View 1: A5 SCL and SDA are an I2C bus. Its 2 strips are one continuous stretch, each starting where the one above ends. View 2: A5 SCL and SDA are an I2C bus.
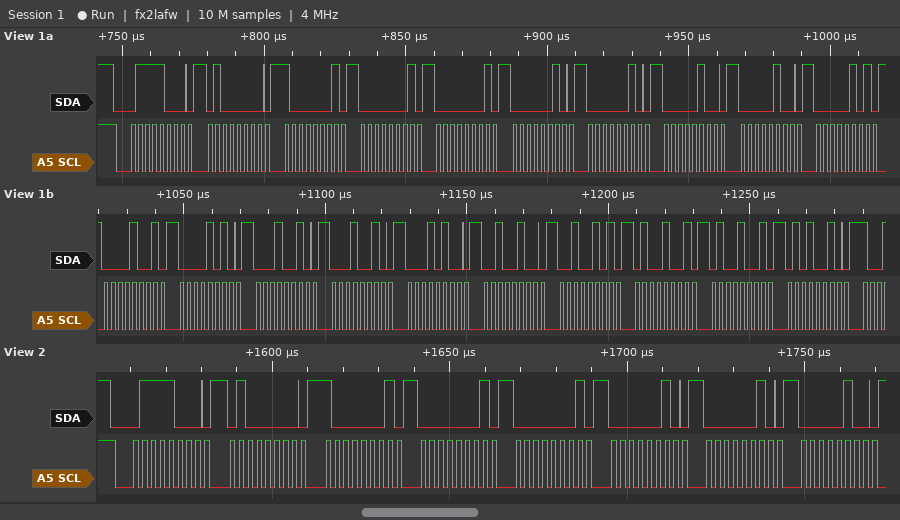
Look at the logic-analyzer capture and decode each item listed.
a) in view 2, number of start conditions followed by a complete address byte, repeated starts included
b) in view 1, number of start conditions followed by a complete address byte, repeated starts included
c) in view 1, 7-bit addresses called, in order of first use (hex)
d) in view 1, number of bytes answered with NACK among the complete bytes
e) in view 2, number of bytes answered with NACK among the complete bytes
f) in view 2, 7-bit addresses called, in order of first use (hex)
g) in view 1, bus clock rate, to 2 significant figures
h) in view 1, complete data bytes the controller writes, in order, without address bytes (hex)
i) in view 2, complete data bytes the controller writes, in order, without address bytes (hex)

1
1
0x3C
0
0
0x3C
400 kHz
40 81 01 01 02 02 04 04 05 09 0A 12 12 14 24 25 49 49 52
40 81 01 01 02 02 04
